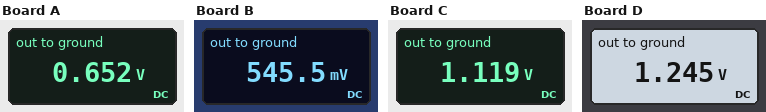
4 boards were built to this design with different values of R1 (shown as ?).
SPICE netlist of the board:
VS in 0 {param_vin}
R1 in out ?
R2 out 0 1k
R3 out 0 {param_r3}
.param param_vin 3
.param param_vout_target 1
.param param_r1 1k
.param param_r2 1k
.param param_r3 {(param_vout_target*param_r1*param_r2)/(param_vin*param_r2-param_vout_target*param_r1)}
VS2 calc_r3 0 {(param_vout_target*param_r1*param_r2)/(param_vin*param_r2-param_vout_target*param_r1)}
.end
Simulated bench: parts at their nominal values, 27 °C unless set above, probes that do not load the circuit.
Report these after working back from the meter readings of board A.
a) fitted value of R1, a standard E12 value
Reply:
1.2 kΩ
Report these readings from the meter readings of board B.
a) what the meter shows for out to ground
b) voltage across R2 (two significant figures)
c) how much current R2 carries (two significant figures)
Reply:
545.5 mV
550 mV
550 µA
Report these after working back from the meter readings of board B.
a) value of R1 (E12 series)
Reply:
1.5 kΩ
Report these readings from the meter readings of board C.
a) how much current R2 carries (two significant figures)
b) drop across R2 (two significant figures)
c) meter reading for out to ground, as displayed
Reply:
1.1 mA
1.1 V
1.119 V
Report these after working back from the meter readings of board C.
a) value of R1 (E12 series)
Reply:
560 Ω
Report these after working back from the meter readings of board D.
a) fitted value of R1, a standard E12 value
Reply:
470 Ω
